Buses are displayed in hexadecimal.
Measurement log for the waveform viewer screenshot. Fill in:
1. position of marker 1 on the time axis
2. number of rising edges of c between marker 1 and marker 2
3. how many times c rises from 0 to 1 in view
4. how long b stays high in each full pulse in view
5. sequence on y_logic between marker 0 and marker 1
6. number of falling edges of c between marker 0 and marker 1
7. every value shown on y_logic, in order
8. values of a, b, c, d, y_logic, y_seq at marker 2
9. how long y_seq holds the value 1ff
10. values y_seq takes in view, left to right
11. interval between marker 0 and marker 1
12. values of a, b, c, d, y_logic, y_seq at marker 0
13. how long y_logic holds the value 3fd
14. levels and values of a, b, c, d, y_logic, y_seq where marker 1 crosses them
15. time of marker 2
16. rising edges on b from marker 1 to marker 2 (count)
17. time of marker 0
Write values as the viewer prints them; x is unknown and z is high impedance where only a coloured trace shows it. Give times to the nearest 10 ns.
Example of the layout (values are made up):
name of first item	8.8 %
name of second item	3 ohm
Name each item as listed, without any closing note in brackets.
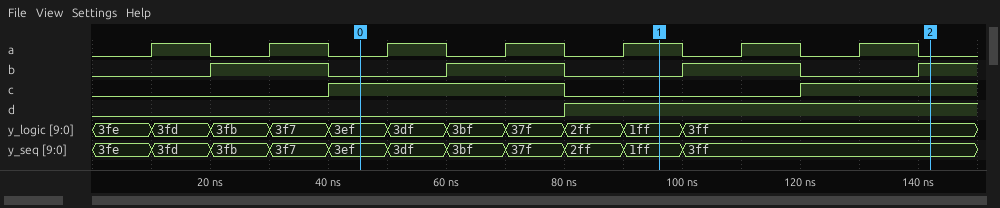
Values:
position of marker 1 on the time axis	100 ns
number of rising edges of c between marker 1 and marker 2	1
how many times c rises from 0 to 1 in view	2
how long b stays high in each full pulse in view	20 ns, 20 ns, 20 ns
sequence on y_logic between marker 0 and marker 1	3ef, 3df, 3bf, 37f, 2ff, 1ff
number of falling edges of c between marker 0 and marker 1	1
every value shown on y_logic, in order	3fe, 3fd, 3fb, 3f7, 3ef, 3df, 3bf, 37f, 2ff, 1ff, 3ff
values of a, b, c, d, y_logic, y_seq at marker 2	a=0, b=1, c=1, d=1, y_logic=3ff, y_seq=3ff
how long y_seq holds the value 1ff	10 ns
values y_seq takes in view, left to right	3fe, 3fd, 3fb, 3f7, 3ef, 3df, 3bf, 37f, 2ff, 1ff, 3ff
interval between marker 0 and marker 1	50 ns
values of a, b, c, d, y_logic, y_seq at marker 0	a=0, b=0, c=1, d=0, y_logic=3ef, y_seq=3ef
how long y_logic holds the value 3fd	10 ns
levels and values of a, b, c, d, y_logic, y_seq where marker 1 crosses them	a=1, b=0, c=0, d=1, y_logic=1ff, y_seq=1ff
time of marker 2	140 ns
rising edges on b from marker 1 to marker 2	2
time of marker 0	50 ns
